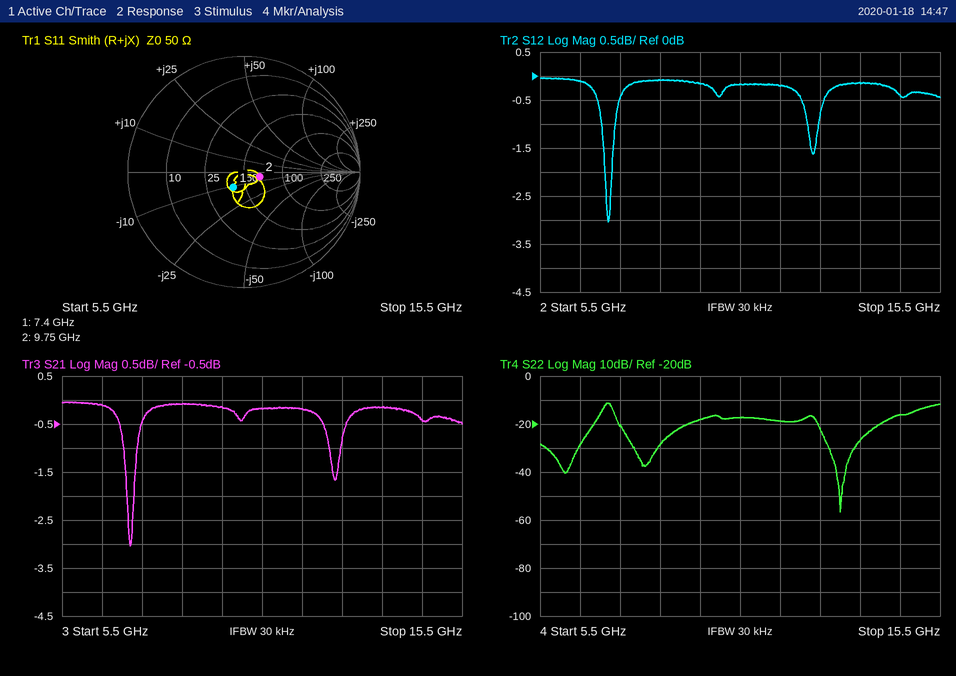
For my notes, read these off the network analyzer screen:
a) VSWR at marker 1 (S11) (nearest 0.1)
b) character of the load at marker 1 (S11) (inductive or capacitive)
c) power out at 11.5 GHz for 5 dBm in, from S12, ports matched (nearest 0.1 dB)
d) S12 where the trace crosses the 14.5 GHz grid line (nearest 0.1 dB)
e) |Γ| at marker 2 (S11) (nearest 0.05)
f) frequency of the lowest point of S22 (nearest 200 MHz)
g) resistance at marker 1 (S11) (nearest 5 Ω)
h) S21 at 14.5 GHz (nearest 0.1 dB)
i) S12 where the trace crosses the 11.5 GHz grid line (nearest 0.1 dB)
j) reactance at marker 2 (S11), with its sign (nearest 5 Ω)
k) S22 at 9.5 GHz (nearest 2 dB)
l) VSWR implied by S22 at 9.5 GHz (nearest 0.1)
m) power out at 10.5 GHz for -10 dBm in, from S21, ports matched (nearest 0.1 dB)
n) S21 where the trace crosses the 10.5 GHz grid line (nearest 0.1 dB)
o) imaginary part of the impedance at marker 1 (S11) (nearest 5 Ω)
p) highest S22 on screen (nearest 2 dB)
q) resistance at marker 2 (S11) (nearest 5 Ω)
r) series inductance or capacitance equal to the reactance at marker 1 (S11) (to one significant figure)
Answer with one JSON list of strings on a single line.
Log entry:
["1.4", "capacitive", "4.8 dBm", "-0.4 dB", "0.15", "13.0 GHz", "40 Ω", "-0.4 dB", "-0.2 dB", "-5 Ω", "-18 dB", "1.3", "-10.2 dBm", "-0.2 dB", "-10 Ω", "-12 dB", "65 Ω", "2 pF"]
